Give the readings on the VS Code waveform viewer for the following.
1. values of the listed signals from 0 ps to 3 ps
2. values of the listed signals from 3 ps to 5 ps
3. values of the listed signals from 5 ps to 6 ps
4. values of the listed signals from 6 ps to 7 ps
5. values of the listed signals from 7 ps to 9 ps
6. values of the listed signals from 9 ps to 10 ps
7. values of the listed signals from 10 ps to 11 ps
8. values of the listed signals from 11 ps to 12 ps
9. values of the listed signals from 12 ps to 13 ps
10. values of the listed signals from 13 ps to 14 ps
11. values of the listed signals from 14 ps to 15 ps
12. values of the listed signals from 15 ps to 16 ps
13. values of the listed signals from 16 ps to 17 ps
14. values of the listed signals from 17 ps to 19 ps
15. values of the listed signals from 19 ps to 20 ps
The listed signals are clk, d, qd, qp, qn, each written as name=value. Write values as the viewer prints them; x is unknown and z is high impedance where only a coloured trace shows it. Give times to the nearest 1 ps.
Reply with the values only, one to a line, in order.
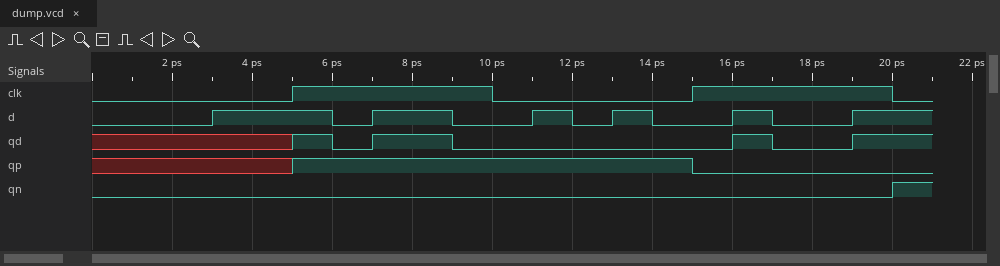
clk=0, d=0, qd=x, qp=x, qn=0
clk=0, d=1, qd=x, qp=x, qn=0
clk=1, d=1, qd=1, qp=1, qn=0
clk=1, d=0, qd=0, qp=1, qn=0
clk=1, d=1, qd=1, qp=1, qn=0
clk=1, d=0, qd=0, qp=1, qn=0
clk=0, d=0, qd=0, qp=1, qn=0
clk=0, d=1, qd=0, qp=1, qn=0
clk=0, d=0, qd=0, qp=1, qn=0
clk=0, d=1, qd=0, qp=1, qn=0
clk=0, d=0, qd=0, qp=1, qn=0
clk=1, d=0, qd=0, qp=0, qn=0
clk=1, d=1, qd=1, qp=0, qn=0
clk=1, d=0, qd=0, qp=0, qn=0
clk=1, d=1, qd=1, qp=0, qn=0
